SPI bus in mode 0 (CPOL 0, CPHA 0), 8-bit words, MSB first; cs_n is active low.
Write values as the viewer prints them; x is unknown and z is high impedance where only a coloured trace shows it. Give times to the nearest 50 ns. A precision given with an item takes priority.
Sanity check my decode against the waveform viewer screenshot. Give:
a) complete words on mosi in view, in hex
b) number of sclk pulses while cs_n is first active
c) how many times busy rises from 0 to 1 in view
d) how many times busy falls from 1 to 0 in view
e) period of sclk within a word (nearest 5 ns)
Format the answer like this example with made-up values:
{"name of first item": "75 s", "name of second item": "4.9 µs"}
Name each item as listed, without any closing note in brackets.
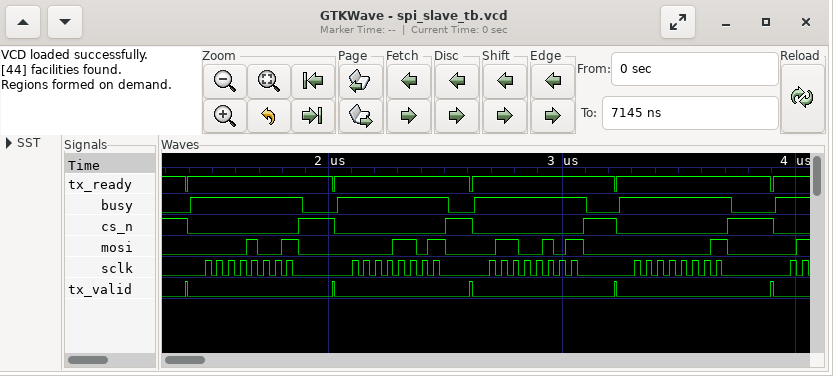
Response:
{"complete words on mosi in view, in hex": "09, 0D, 65, 01", "number of sclk pulses while cs_n is first active": "8", "how many times busy rises from 0 to 1 in view": "5", "how many times busy falls from 1 to 0 in view": "4", "period of sclk within a word": "50 ns"}
